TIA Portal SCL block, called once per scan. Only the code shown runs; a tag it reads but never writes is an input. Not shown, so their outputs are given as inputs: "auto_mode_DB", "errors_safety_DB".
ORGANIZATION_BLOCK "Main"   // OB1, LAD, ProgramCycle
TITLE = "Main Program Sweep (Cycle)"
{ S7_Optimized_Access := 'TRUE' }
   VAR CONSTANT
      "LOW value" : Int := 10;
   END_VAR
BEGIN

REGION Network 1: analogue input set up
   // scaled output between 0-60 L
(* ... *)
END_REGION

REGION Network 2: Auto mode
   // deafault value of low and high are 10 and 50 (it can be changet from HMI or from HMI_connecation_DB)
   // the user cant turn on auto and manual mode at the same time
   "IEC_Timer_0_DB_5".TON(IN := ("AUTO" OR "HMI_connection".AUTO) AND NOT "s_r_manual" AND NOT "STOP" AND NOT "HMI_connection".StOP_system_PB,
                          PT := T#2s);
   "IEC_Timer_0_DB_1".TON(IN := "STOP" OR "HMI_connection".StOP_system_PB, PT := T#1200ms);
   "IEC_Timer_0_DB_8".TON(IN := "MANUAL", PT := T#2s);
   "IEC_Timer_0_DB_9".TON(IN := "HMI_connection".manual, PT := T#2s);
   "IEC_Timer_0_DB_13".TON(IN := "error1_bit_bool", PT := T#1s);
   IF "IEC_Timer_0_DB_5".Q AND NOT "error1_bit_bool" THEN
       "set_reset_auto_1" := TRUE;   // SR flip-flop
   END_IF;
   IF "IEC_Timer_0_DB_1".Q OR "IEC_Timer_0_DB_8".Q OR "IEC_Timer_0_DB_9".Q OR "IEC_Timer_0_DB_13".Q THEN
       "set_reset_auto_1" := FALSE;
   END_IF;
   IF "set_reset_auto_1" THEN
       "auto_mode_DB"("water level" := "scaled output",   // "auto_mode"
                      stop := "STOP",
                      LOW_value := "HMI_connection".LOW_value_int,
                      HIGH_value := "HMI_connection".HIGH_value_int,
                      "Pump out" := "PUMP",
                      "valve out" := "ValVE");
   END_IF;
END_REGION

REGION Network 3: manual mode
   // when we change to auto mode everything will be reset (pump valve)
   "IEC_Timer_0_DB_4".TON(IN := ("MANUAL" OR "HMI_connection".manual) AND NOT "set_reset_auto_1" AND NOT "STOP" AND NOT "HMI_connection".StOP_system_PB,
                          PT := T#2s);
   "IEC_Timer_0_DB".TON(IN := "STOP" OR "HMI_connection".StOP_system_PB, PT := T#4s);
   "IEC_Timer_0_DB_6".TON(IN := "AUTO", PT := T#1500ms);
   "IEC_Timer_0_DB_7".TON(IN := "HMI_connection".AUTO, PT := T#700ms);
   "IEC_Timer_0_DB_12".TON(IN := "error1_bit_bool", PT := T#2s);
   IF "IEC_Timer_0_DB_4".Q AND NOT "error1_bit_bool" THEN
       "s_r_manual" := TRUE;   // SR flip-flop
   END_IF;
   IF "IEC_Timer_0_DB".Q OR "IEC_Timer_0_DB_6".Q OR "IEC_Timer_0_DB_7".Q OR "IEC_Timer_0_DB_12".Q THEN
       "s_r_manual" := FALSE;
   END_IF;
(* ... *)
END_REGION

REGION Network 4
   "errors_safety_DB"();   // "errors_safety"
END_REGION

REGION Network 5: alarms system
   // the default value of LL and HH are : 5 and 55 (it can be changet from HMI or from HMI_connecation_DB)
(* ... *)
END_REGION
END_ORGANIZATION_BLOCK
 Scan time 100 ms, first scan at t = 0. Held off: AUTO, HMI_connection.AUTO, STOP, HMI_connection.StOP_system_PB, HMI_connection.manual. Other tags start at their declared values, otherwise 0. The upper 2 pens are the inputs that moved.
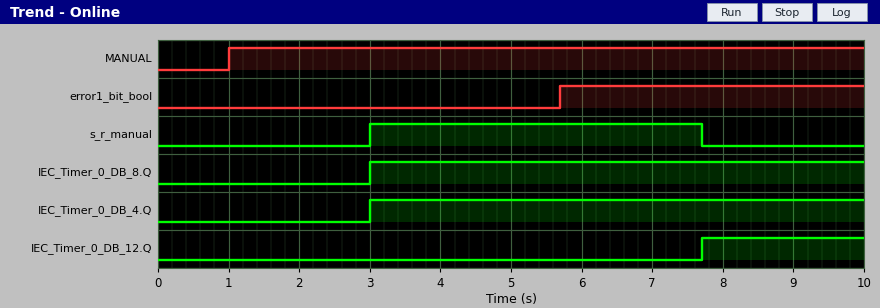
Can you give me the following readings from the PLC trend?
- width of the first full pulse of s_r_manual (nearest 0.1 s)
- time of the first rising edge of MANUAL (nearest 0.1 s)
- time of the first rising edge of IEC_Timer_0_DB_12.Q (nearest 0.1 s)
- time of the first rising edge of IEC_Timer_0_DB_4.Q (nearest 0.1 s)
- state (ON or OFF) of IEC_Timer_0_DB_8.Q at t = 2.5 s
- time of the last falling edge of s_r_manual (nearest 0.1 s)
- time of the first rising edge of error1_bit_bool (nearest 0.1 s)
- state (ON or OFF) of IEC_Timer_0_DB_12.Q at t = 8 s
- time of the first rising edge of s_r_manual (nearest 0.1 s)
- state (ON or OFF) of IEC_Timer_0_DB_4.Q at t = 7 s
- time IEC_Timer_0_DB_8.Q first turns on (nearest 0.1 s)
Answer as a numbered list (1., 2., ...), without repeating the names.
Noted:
1. 4.7 s
2. 1.0 s
3. 7.7 s
4. 3.0 s
5. OFF
6. 7.7 s
7. 5.7 s
8. ON
9. 3.0 s
10. ON
11. 3.0 s
